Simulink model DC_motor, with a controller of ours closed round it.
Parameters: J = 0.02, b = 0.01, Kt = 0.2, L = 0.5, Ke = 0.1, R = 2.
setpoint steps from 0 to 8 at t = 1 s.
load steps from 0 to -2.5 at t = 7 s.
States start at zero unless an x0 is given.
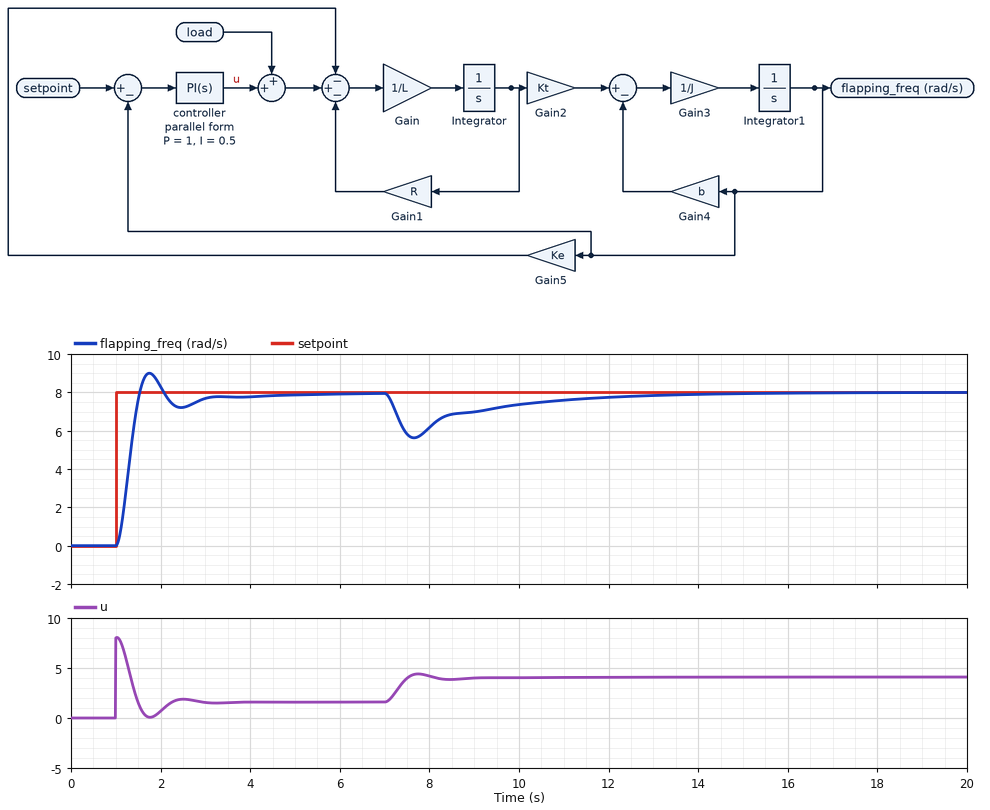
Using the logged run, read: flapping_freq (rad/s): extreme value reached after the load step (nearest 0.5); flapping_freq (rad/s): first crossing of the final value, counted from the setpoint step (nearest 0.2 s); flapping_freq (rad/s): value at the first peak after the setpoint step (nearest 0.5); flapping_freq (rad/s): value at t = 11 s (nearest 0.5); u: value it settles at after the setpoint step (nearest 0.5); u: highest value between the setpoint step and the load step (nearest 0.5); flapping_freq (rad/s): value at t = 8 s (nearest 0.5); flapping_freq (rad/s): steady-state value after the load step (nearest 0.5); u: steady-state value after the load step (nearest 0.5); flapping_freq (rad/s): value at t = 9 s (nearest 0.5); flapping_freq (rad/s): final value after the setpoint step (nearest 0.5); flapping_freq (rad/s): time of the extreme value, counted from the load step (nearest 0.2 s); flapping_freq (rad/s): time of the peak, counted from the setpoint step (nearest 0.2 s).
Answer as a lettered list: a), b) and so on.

a) 5.5
b) 0.6 s
c) 9.0
d) 7.5
e) 1.5
f) 8.0
g) 6.0
h) 8.0
i) 4.0
j) 7.0
k) 8.0
l) 0.6 s
m) 0.8 s
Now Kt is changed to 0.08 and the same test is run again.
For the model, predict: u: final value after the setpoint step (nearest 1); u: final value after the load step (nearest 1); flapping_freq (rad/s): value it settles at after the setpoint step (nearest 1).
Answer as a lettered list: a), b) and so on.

a) 3
b) 5
c) 8
